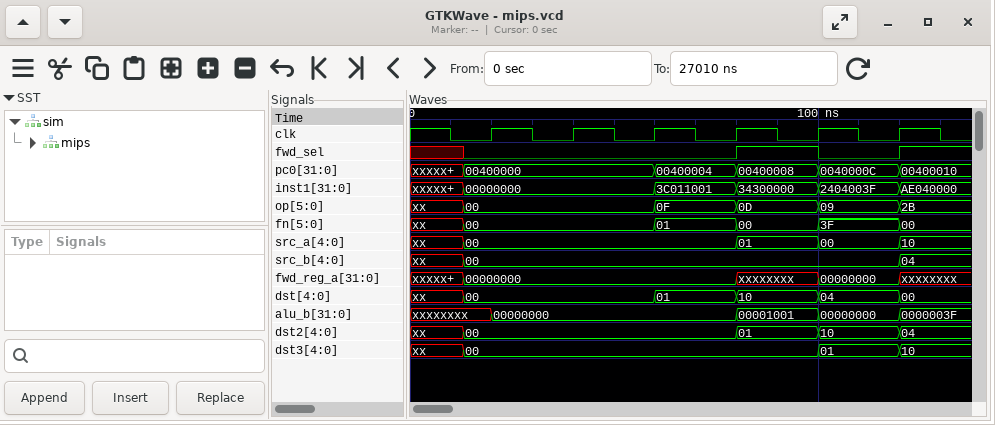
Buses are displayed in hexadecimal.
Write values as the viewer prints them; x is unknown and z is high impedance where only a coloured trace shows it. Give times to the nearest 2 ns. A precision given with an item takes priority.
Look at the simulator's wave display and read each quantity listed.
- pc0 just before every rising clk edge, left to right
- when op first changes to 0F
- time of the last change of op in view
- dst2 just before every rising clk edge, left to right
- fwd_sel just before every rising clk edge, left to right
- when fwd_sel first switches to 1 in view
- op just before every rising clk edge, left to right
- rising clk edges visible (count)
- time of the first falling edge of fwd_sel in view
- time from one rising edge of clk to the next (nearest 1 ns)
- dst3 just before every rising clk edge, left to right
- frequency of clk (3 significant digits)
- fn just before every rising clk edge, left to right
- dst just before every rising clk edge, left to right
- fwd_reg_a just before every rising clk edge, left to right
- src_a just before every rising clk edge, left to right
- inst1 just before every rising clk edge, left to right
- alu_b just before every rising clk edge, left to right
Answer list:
00400000, 00400000, 00400000, 00400004, 00400008, 0040000C
60 ns
120 ns
00, 00, 00, 00, 01, 10
0 0 0 0 1 0
80 ns
00, 00, 00, 0F, 0D, 09
6
100 ns
20 ns
00, 00, 00, 00, 00, 01
50.0 MHz
00, 00, 00, 01, 00, 3F
00, 00, 00, 01, 10, 04
00000000, 00000000, 00000000, 00000000, xxxxxxxx, 00000000
00, 00, 00, 00, 01, 00
00000000, 00000000, 00000000, 3C011001, 34300000, 2404003F
xxxxxxxx, 00000000, 00000000, 00000000, 00001001, 00000000
